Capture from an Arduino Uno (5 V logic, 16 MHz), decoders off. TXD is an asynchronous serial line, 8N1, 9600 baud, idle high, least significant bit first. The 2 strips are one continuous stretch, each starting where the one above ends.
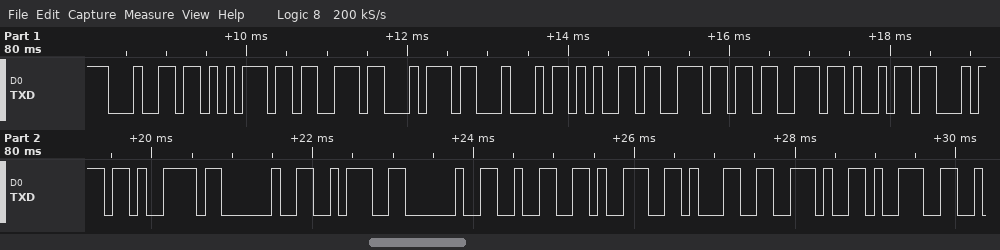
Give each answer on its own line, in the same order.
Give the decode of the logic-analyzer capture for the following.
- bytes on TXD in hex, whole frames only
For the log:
0x64 0x75 0x73 0x74 0x44 0x65 0x6E 0x73 0x69 0x74 0x79 0x20 0x3A 0x20 0x32 0x39 0x31 0x2E 0x39
